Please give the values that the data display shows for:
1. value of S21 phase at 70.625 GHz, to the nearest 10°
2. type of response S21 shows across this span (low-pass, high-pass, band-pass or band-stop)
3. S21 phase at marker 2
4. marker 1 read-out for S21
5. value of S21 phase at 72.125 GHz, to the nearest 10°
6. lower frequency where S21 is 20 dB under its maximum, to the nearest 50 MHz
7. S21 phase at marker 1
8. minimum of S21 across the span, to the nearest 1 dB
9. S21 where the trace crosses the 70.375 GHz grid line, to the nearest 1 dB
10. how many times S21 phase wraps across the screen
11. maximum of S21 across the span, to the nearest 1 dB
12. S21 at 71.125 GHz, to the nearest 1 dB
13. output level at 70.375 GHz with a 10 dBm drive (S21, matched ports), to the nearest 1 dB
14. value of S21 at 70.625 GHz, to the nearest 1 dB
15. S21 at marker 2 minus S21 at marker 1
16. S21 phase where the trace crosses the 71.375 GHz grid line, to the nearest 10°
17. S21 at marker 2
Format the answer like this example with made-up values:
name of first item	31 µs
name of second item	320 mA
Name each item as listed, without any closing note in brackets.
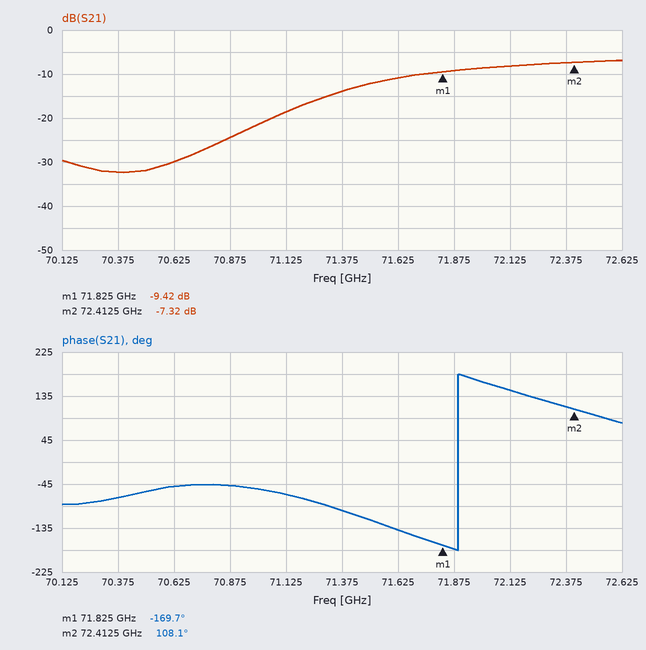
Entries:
value of S21 phase at 70.625 GHz, to the nearest 10°	-50°
type of response S21 shows across this span	high-pass
S21 phase at marker 2	108.1°
marker 1 read-out for S21	-9.42 dB
value of S21 phase at 72.125 GHz, to the nearest 10°	150°
lower frequency where S21 is 20 dB under its maximum, to the nearest 50 MHz	70.75 GHz
S21 phase at marker 1	-169.7°
minimum of S21 across the span, to the nearest 1 dB	-32 dB
S21 where the trace crosses the 70.375 GHz grid line, to the nearest 1 dB	-32 dB
how many times S21 phase wraps across the screen	1
maximum of S21 across the span, to the nearest 1 dB	-7 dB
S21 at 71.125 GHz, to the nearest 1 dB	-19 dB
output level at 70.375 GHz with a 10 dBm drive (S21, matched ports), to the nearest 1 dB	-22 dBm
value of S21 at 70.625 GHz, to the nearest 1 dB	-30 dB
S21 at marker 2 minus S21 at marker 1	2.10 dB
S21 phase where the trace crosses the 71.375 GHz grid line, to the nearest 10°	-100°
S21 at marker 2	-7.32 dB
